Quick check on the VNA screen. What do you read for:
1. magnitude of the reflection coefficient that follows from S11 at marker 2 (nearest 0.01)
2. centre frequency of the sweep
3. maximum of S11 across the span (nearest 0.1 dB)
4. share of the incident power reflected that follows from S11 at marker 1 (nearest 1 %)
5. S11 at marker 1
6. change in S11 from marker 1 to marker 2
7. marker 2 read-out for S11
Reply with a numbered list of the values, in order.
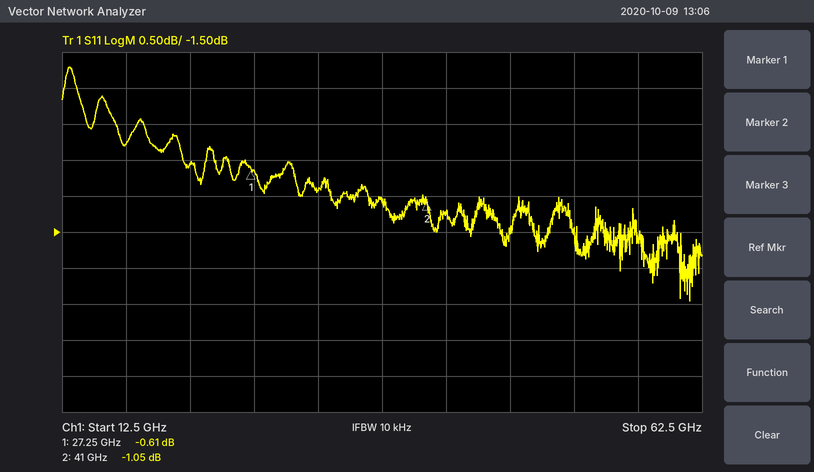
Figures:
1. 0.89
2. 37.5 GHz
3. 0.8 dB
4. 87 %
5. -0.61 dB
6. -0.44 dB
7. -1.05 dB
